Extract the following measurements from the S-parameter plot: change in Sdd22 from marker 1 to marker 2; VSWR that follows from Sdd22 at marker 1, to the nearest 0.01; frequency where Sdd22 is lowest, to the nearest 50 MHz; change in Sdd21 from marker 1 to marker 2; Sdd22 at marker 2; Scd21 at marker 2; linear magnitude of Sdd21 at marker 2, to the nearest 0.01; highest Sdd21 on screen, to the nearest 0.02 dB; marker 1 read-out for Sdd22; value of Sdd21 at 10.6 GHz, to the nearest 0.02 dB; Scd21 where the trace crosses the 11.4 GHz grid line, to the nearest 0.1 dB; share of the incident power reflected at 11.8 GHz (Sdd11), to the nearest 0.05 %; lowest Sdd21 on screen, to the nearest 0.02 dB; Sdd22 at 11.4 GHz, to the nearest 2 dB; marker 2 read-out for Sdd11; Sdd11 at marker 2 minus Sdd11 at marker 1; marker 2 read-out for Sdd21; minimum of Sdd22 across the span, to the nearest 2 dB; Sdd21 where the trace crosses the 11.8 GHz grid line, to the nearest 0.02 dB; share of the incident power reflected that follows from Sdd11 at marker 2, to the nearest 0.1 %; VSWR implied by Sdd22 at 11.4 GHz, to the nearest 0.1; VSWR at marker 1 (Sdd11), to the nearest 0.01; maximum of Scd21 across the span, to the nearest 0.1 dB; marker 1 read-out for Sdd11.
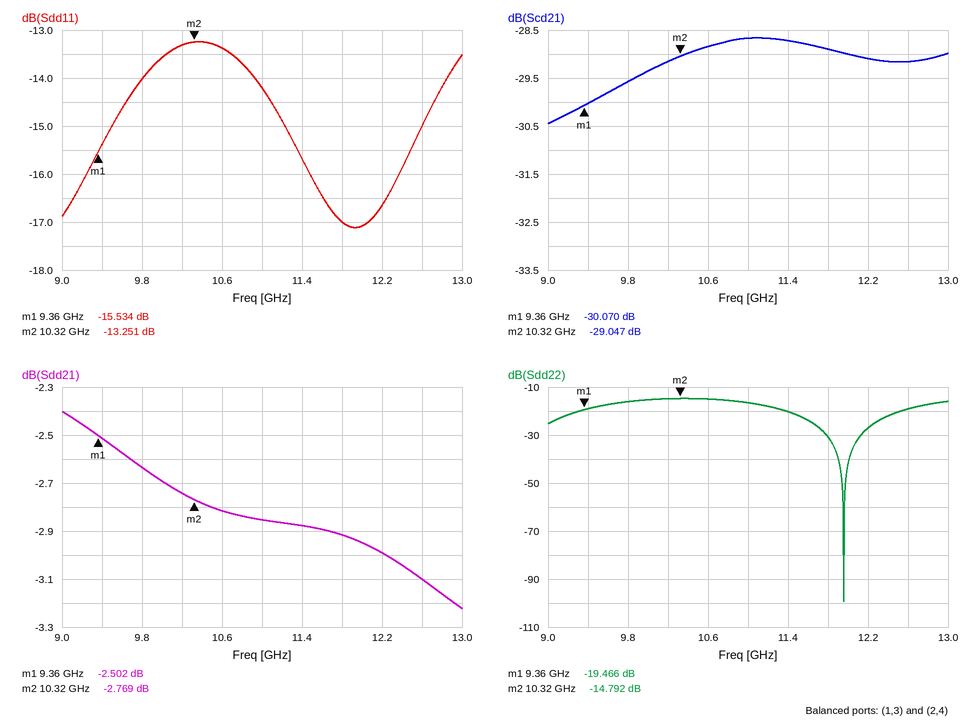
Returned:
4.674 dB
1.24
11.95 GHz
-0.267 dB
-14.792 dB
-29.047 dB
0.73
-2.40 dB
-19.466 dB
-2.82 dB
-28.7 dB
2.00 %
-3.22 dB
-20 dB
-13.251 dB
2.283 dB
-2.769 dB
-100 dB
-2.92 dB
4.7 %
1.2
1.40
-28.7 dB
-15.534 dB
